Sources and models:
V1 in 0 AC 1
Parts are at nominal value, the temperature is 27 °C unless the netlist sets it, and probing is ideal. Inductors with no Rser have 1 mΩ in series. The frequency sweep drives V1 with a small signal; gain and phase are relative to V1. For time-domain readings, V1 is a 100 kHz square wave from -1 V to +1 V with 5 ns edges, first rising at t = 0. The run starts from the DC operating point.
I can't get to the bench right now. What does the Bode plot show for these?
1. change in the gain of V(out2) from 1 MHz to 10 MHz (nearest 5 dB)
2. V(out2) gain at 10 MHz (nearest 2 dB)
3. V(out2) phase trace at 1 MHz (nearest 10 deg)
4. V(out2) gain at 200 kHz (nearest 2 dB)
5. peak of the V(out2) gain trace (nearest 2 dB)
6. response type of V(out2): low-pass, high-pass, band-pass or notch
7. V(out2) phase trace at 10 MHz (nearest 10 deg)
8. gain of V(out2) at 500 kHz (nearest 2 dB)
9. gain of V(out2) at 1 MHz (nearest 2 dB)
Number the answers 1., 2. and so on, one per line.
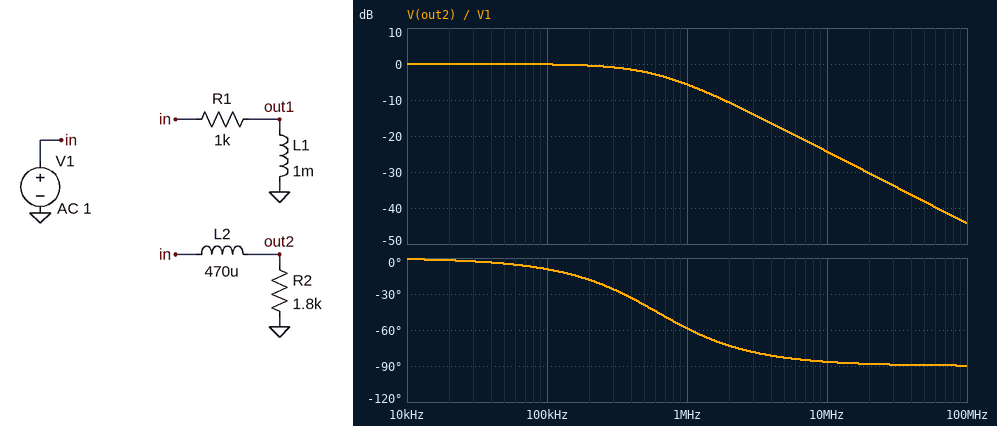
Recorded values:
1. -20 dB
2. -24 dB
3. -60 deg
4. 0 dB
5. 0 dB
6. low-pass
7. -90 deg
8. -2 dB
9. -6 dB
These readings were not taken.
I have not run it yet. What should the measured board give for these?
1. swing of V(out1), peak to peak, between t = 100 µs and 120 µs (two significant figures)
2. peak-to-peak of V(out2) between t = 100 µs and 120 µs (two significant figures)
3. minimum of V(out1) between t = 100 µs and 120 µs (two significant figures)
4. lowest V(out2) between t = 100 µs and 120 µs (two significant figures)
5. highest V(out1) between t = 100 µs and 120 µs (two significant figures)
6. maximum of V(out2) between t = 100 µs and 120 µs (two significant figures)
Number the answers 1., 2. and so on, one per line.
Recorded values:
1. 4.0 V
2. 2.0 V
3. -2.0 V
4. -1.0 V
5. 2.0 V
6. 1.0 V
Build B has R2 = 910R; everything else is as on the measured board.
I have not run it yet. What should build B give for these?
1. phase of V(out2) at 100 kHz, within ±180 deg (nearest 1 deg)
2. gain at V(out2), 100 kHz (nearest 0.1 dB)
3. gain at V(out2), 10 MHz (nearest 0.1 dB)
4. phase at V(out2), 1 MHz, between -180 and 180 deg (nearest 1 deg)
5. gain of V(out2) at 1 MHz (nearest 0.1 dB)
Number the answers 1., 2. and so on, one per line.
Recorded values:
1. -18 deg
2. -0.4 dB
3. -30.2 dB
4. -73 deg
5. -10.6 dB
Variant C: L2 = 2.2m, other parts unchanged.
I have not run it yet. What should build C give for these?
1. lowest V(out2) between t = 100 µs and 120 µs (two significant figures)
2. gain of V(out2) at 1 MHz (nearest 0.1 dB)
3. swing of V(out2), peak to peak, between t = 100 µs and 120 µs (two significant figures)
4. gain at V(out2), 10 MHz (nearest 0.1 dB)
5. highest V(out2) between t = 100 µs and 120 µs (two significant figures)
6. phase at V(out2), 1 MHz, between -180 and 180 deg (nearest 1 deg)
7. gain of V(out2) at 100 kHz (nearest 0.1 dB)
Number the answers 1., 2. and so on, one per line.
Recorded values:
1. -970 mV
2. -17.8 dB
3. 1.9 V
4. -37.7 dB
5. 970 mV
6. -83 deg
7. -2.0 dB
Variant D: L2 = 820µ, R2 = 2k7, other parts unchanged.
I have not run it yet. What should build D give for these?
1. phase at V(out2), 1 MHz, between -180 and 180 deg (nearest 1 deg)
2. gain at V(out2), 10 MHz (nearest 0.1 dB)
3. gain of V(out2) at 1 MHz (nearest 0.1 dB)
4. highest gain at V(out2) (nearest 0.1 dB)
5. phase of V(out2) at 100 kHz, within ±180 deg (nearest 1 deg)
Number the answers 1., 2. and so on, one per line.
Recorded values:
1. -62 deg
2. -25.6 dB
3. -6.7 dB
4. 0 dB
5. -11 deg
